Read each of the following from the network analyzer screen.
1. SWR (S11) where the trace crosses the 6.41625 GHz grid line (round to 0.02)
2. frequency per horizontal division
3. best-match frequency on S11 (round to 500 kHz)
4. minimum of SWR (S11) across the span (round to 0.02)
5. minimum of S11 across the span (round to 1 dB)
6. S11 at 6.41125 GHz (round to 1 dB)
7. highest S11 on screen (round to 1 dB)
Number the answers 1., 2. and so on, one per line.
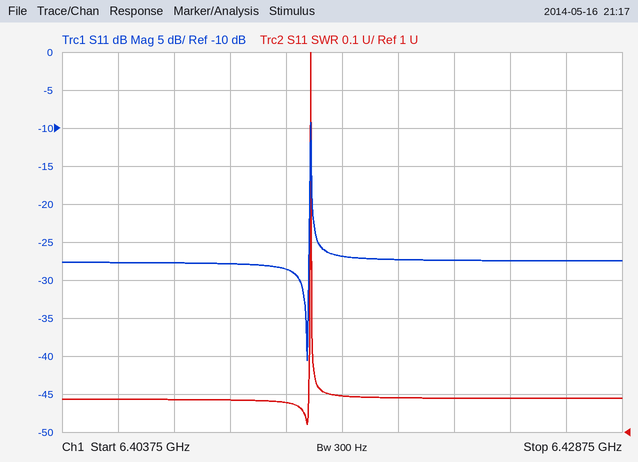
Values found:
1. 1.10
2. 2.5 MHz
3. 6.4145 GHz
4. 1.02
5. -41 dB
6. -28 dB
7. -9 dB
